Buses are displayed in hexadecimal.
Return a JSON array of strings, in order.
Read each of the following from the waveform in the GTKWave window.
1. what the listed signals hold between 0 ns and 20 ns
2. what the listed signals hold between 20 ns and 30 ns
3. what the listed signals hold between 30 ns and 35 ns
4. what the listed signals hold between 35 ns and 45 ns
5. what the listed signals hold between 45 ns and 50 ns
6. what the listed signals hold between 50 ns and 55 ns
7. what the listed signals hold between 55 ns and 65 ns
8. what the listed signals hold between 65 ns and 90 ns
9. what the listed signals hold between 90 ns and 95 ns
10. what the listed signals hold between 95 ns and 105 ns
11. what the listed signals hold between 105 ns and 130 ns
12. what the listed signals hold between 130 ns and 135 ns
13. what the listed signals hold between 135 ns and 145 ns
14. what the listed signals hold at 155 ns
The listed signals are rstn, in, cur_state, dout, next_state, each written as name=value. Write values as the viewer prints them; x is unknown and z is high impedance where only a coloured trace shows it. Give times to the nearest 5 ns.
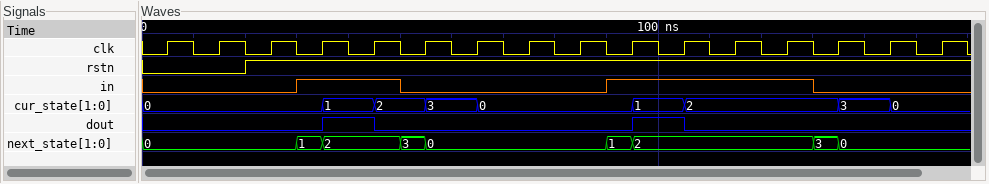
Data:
["rstn=0, in=0, cur_state=0, dout=0, next_state=0", "rstn=1, in=0, cur_state=0, dout=0, next_state=0", "rstn=1, in=1, cur_state=0, dout=0, next_state=1", "rstn=1, in=1, cur_state=1, dout=1, next_state=2", "rstn=1, in=1, cur_state=2, dout=0, next_state=2", "rstn=1, in=0, cur_state=2, dout=0, next_state=3", "rstn=1, in=0, cur_state=3, dout=0, next_state=0", "rstn=1, in=0, cur_state=0, dout=0, next_state=0", "rstn=1, in=1, cur_state=0, dout=0, next_state=1", "rstn=1, in=1, cur_state=1, dout=1, next_state=2", "rstn=1, in=1, cur_state=2, dout=0, next_state=2", "rstn=1, in=0, cur_state=2, dout=0, next_state=3", "rstn=1, in=0, cur_state=3, dout=0, next_state=0", "rstn=1, in=0, cur_state=0, dout=0, next_state=0"]
